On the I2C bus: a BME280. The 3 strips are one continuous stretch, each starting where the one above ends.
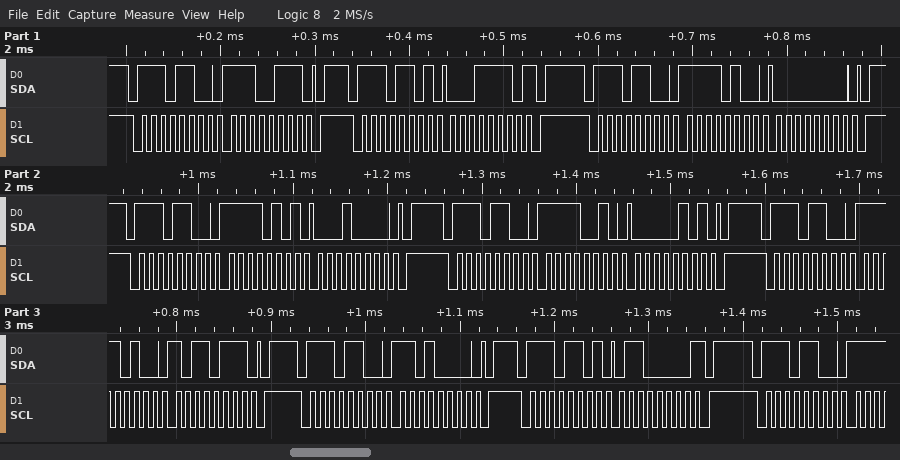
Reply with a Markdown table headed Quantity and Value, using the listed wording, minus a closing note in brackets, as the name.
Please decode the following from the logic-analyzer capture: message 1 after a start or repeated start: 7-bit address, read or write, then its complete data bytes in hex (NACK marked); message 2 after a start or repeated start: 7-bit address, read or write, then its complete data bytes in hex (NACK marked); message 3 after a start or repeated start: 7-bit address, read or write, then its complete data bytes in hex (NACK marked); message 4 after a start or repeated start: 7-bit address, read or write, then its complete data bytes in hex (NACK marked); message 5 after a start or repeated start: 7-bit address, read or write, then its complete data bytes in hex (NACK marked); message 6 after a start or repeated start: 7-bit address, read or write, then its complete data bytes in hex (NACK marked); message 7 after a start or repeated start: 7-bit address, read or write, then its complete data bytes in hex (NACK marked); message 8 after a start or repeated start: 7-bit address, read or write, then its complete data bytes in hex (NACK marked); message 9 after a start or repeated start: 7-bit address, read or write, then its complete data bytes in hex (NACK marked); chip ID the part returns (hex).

| Quantity | Value |
|---|---|
| message 1 after a start or repeated start: 7-bit address, read or write, then its complete data bytes in hex | 0x76 write: E7 |
| message 2 after a start or repeated start: 7-bit address, read or write, then its complete data bytes in hex | 0x76 read: 1E NACK |
| message 3 after a start or repeated start: 7-bit address, read or write, then its complete data bytes in hex | 0x76 write: F4 00 |
| message 4 after a start or repeated start: 7-bit address, read or write, then its complete data bytes in hex | 0x76 write: F5 10 |
| message 5 after a start or repeated start: 7-bit address, read or write, then its complete data bytes in hex | 0x76 write: F2 05 |
| message 6 after a start or repeated start: 7-bit address, read or write, then its complete data bytes in hex | 0x76 write: F4 B7 |
| message 7 after a start or repeated start: 7-bit address, read or write, then its complete data bytes in hex | 0x76 write: D0 |
| message 8 after a start or repeated start: 7-bit address, read or write, then its complete data bytes in hex | 0x76 read: 60 NACK |
| message 9 after a start or repeated start: 7-bit address, read or write, then its complete data bytes in hex | 0x76 write |
| chip ID the part returns | 0x60 |
